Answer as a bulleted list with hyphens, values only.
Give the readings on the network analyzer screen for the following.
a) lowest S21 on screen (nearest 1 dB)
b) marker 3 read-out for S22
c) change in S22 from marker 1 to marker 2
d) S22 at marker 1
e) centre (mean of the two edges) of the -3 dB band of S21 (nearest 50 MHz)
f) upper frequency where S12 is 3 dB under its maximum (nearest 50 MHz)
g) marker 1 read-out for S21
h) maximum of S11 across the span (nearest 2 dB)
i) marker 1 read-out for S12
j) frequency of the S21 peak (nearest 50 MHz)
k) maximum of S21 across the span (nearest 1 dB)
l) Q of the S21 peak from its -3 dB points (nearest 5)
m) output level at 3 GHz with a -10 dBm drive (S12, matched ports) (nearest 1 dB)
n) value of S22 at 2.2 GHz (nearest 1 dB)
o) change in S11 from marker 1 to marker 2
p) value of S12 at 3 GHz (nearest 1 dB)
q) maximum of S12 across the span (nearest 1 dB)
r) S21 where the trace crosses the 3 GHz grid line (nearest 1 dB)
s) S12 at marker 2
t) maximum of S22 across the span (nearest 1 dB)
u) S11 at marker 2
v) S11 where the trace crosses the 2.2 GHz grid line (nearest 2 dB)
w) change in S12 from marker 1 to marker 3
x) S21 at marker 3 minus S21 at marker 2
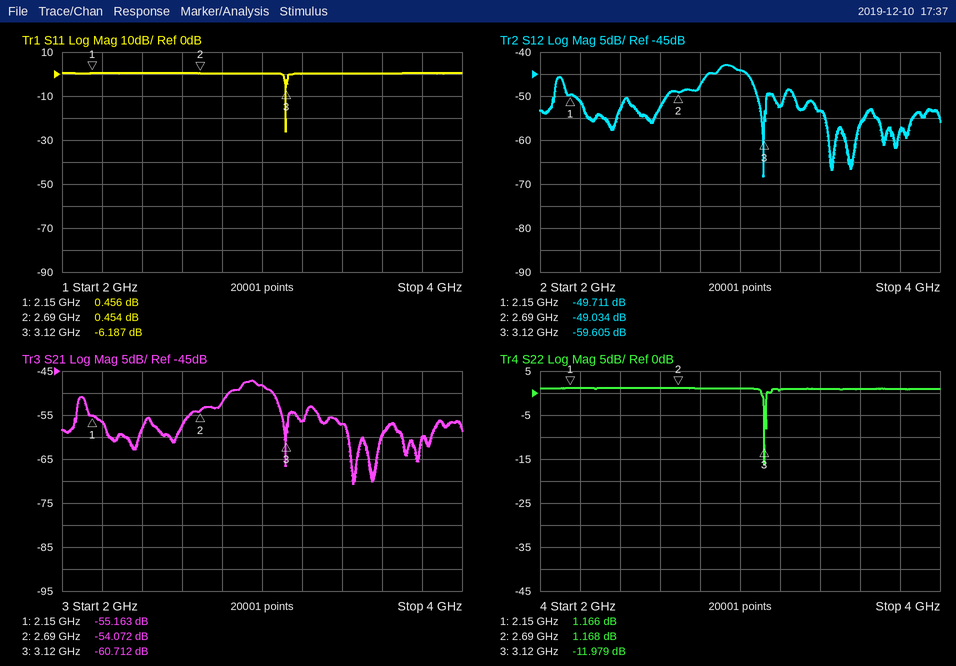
- -71 dB
- -11.979 dB
- 0.002 dB
- 1.166 dB
- 2.95 GHz
- 3.05 GHz
- -55.163 dB
- 0 dB
- -49.711 dB
- 2.95 GHz
- -47 dB
- 15
- -54 dBm
- 1 dB
- -0.002 dB
- -44 dB
- -43 dB
- -48 dB
- -49.034 dB
- 1 dB
- 0.454 dB
- 0 dB
- -9.894 dB
- -6.640 dB
